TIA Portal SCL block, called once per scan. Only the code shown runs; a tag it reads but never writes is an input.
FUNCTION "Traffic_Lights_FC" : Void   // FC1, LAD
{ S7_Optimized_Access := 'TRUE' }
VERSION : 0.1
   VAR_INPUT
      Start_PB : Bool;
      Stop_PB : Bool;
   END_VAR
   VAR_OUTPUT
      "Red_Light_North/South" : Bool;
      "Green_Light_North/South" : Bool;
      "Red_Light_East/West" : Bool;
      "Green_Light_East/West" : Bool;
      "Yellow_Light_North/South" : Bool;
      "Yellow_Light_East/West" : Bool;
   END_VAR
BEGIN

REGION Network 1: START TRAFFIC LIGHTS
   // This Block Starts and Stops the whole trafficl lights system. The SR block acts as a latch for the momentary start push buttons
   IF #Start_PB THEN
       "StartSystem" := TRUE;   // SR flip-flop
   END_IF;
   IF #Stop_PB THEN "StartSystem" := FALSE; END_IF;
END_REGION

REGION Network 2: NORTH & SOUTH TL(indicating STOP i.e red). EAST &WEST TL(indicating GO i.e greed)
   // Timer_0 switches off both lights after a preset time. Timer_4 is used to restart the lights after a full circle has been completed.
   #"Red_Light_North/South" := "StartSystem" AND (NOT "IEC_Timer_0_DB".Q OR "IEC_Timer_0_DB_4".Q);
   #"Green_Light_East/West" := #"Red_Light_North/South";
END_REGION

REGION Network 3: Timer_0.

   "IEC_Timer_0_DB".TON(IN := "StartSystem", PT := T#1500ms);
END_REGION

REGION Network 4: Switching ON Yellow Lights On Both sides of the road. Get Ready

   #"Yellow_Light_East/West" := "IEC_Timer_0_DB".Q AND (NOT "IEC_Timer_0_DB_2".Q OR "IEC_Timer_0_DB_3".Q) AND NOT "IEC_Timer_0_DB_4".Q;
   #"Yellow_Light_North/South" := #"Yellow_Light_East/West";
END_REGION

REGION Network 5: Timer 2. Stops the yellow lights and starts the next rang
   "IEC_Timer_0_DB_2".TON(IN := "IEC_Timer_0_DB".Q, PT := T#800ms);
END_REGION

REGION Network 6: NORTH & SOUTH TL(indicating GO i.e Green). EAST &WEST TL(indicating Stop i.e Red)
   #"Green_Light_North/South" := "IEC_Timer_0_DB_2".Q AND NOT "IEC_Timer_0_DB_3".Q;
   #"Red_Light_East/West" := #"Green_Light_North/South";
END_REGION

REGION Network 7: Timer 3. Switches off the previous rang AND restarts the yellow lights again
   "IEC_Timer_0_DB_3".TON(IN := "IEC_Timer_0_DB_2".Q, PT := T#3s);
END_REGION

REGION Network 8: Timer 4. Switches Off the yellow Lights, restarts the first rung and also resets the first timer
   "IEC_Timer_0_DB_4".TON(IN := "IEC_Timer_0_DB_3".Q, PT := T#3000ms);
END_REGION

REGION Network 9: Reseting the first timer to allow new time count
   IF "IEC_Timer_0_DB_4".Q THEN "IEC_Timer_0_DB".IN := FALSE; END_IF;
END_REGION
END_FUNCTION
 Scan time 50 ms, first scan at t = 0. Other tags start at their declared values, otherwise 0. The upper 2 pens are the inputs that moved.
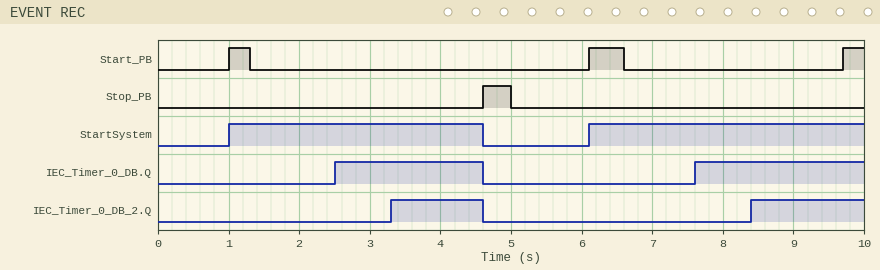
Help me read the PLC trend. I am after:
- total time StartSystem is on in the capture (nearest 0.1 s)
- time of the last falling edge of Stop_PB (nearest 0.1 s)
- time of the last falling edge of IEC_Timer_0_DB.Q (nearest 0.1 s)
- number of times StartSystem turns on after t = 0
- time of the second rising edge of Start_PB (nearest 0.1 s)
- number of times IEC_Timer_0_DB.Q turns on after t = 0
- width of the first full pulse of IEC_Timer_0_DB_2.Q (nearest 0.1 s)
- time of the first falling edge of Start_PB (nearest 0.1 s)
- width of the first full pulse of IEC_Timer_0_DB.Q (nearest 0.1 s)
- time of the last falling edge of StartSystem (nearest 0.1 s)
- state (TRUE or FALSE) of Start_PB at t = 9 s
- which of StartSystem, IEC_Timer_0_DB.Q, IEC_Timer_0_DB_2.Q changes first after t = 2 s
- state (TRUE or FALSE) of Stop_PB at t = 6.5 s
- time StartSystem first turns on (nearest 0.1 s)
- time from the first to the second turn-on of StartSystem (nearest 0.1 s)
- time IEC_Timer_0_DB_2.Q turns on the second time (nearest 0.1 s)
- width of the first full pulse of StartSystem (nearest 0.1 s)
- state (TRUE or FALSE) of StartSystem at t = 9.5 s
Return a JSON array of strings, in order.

["7.5 s", "5.0 s", "4.6 s", "2", "6.1 s", "2", "1.3 s", "1.3 s", "2.1 s", "4.6 s", "FALSE", "IEC_Timer_0_DB.Q", "FALSE", "1.0 s", "5.1 s", "8.4 s", "3.6 s", "TRUE"]
